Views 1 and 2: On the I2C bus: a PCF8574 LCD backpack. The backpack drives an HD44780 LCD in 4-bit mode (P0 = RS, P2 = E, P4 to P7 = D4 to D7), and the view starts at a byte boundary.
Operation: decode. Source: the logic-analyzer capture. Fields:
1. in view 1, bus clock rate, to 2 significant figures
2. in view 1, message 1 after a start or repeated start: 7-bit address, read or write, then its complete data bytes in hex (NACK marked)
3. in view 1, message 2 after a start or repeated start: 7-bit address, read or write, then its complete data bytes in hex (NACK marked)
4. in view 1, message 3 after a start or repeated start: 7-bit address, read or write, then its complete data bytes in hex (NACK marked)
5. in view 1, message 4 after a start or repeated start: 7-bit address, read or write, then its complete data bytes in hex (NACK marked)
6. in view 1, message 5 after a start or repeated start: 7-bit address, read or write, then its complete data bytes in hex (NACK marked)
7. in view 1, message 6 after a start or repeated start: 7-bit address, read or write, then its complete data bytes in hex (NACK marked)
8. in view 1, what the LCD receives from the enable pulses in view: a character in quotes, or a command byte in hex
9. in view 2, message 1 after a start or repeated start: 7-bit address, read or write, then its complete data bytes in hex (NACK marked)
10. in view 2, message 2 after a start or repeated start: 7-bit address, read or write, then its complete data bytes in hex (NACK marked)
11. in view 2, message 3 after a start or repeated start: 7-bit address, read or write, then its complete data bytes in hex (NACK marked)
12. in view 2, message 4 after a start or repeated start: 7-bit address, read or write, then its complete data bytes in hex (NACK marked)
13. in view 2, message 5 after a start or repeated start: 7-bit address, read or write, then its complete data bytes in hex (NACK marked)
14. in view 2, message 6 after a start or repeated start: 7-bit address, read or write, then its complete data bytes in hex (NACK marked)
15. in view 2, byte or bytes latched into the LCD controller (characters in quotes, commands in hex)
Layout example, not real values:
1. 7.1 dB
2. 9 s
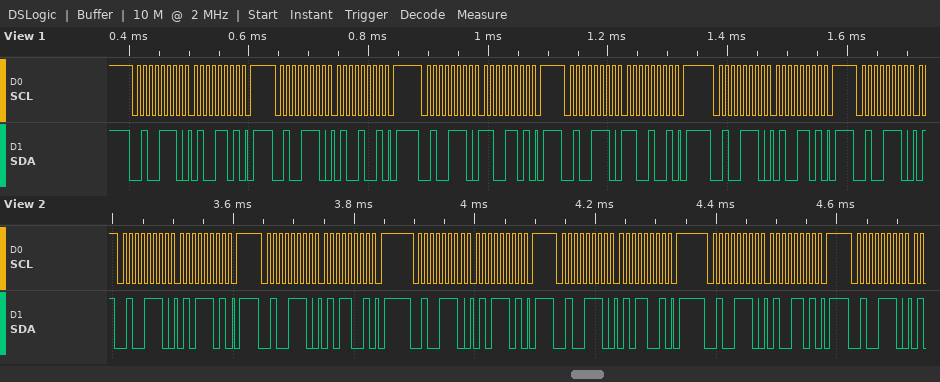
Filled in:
1. 100 kHz
2. 0x27 write: 4D
3. 0x27 write: 49
4. 0x27 write: CD
5. 0x27 write: C9
6. 0x27 write: 4D
7. 0x27 write
8. 'L'
9. 0x27 write: 5D
10. 0x27 write: 59
11. 0x27 write: 5D
12. 0x27 write: 59
13. 0x27 write: 4D
14. 0x27 write
15. 'U'
